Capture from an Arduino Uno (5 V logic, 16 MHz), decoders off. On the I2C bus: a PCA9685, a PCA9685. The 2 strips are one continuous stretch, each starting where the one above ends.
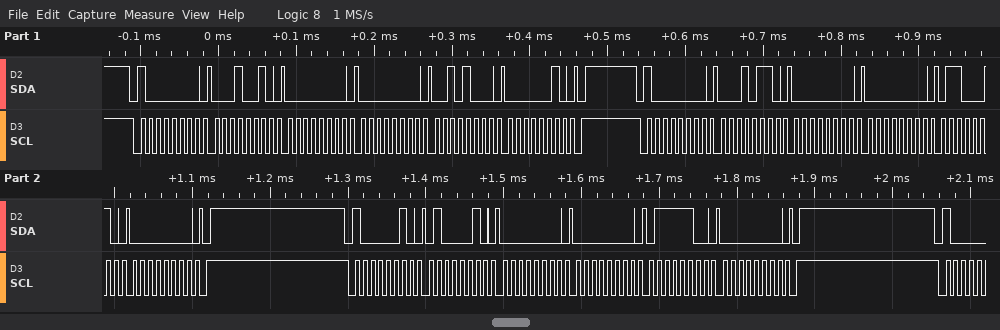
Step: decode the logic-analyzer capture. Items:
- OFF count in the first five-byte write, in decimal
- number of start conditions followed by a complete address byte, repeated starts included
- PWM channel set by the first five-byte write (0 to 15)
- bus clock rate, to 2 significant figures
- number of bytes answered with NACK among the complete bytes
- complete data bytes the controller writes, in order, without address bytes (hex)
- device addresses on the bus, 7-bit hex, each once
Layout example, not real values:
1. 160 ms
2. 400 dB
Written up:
1. 552
2. 3
3. 3
4. 100 kHz
5. 0
6. 12 00 00 28 02 16 00 00 62 00 42 00 00 7C 00
7. 0x40 0x41
